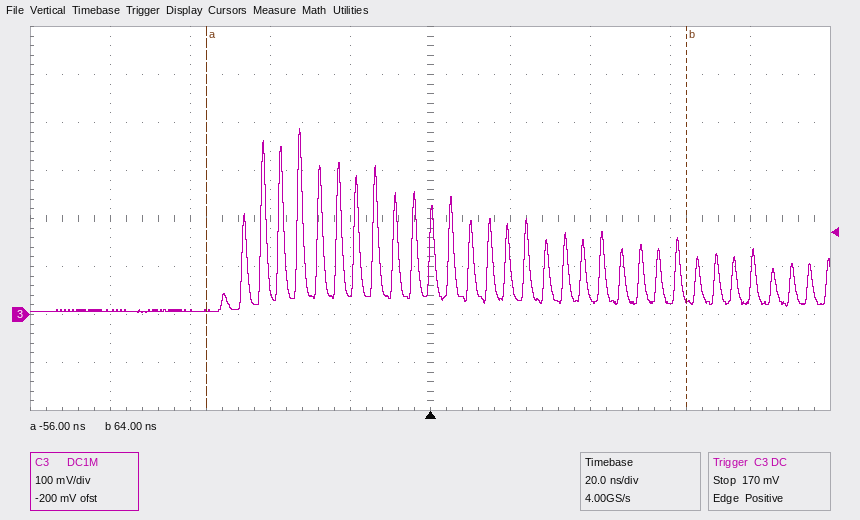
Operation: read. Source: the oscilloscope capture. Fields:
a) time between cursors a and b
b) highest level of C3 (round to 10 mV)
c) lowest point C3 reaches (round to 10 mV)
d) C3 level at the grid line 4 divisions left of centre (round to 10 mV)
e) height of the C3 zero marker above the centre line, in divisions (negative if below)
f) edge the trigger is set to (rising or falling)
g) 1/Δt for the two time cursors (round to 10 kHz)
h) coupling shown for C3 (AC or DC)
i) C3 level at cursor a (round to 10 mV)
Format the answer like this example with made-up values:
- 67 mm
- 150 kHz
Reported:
- 120 ns
- 390 mV
- 0 mV
- 10 mV
- -2.0 div
- rising
- 8.33 MHz
- DC
- 10 mV
